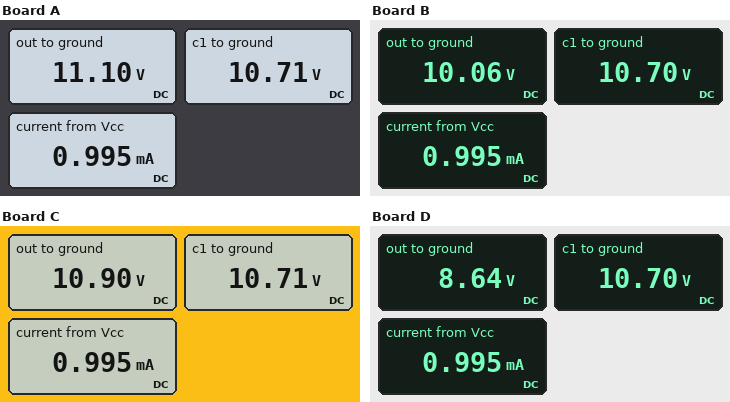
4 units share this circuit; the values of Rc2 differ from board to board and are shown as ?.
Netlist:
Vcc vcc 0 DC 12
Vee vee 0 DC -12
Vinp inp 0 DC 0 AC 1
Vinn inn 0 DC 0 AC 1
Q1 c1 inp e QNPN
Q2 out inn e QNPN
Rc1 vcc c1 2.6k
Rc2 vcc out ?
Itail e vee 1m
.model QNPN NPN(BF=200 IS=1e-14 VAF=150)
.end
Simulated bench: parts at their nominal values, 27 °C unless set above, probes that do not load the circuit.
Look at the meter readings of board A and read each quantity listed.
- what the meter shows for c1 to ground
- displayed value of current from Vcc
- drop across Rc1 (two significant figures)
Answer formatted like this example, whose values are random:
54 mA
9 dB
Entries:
10.71 V
0.995 mA
1.3 V
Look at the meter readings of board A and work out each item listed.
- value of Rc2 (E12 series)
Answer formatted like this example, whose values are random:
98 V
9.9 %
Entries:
1.8 kΩ
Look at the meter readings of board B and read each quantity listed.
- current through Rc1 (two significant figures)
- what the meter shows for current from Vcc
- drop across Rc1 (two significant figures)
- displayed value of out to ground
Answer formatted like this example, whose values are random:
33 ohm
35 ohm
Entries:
500 µA
0.995 mA
1.3 V
10.06 V
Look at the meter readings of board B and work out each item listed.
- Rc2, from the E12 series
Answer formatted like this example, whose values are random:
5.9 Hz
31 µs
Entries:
3.9 kΩ
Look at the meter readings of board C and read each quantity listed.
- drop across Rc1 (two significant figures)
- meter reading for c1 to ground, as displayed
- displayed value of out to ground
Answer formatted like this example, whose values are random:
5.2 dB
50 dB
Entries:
1.3 V
10.71 V
10.90 V
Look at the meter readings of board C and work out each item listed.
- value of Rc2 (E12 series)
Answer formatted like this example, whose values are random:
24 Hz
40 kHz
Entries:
2.2 kΩ
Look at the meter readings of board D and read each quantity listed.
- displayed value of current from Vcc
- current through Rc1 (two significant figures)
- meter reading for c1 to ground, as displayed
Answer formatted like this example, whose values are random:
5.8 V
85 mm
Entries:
0.995 mA
500 µA
10.70 V
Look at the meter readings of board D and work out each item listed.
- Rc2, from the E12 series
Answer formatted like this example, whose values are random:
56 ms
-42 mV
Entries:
6.8 kΩ
